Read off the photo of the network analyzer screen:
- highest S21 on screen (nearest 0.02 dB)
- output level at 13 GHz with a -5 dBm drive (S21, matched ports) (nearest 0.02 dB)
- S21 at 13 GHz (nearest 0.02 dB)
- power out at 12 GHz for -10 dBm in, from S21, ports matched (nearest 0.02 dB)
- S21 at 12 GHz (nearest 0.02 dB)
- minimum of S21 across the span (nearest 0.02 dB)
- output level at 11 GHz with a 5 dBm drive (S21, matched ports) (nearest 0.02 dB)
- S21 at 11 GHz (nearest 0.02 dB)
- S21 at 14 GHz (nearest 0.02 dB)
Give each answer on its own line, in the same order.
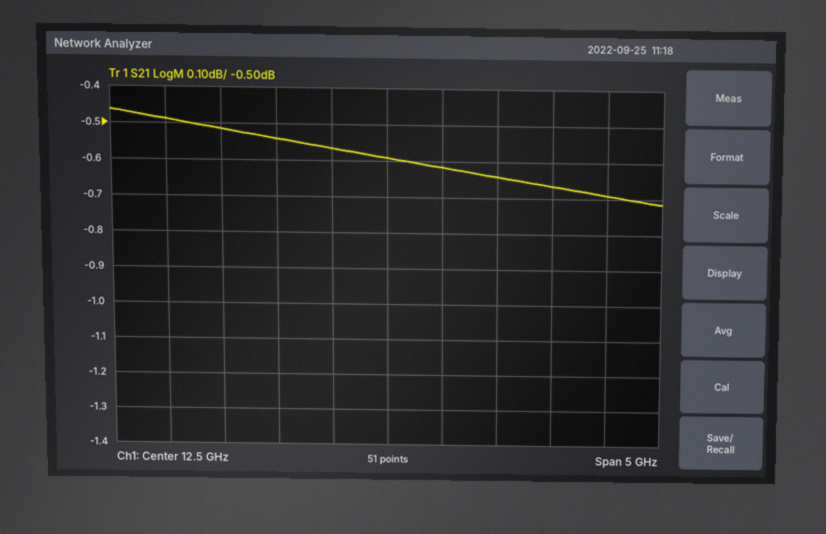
-0.46 dB
-5.62 dBm
-0.62 dB
-10.56 dBm
-0.56 dB
-0.72 dB
4.48 dBm
-0.52 dB
-0.66 dB
